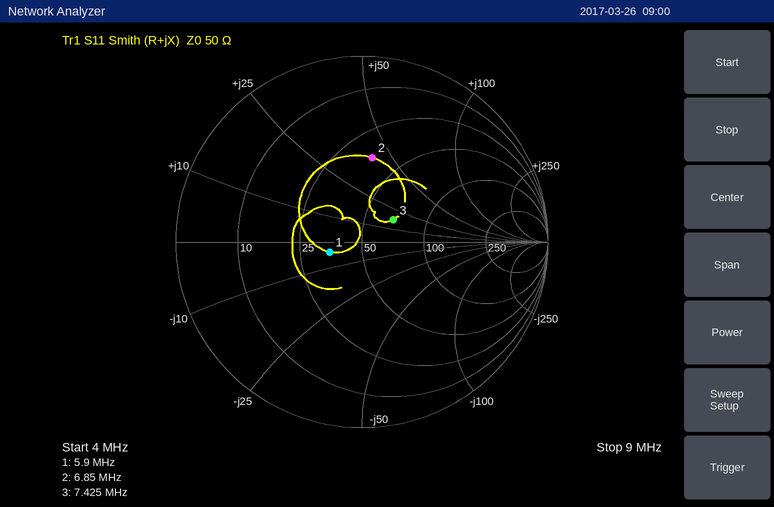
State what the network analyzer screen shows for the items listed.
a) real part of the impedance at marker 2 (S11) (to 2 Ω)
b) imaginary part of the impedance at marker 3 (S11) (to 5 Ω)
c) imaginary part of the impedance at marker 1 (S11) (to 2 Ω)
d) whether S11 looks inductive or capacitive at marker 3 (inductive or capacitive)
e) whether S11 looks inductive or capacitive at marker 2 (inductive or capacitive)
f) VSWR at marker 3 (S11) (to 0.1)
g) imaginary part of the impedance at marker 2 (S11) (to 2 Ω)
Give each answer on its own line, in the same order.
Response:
36 Ω
+15 Ω
-4 Ω
inductive
inductive
1.5
+42 Ω
